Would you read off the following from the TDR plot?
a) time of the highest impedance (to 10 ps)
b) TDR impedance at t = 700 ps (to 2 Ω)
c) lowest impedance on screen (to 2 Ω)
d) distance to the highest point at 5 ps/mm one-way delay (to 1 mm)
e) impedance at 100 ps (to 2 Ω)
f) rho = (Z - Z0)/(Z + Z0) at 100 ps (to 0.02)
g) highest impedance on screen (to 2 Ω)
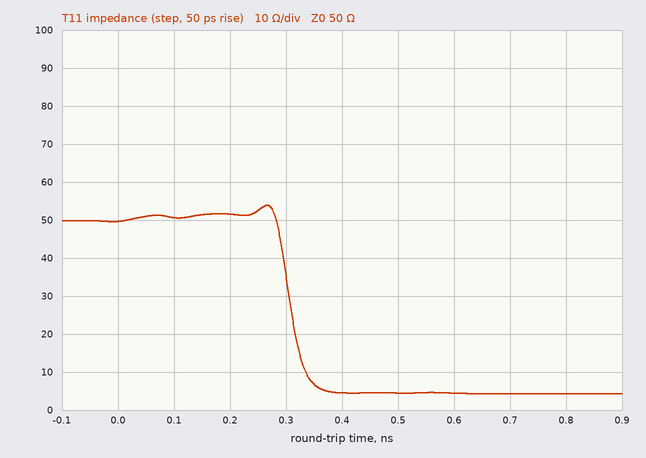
270 ps
4 Ω
4 Ω
27 mm
50 Ω
0.00
54 Ω
